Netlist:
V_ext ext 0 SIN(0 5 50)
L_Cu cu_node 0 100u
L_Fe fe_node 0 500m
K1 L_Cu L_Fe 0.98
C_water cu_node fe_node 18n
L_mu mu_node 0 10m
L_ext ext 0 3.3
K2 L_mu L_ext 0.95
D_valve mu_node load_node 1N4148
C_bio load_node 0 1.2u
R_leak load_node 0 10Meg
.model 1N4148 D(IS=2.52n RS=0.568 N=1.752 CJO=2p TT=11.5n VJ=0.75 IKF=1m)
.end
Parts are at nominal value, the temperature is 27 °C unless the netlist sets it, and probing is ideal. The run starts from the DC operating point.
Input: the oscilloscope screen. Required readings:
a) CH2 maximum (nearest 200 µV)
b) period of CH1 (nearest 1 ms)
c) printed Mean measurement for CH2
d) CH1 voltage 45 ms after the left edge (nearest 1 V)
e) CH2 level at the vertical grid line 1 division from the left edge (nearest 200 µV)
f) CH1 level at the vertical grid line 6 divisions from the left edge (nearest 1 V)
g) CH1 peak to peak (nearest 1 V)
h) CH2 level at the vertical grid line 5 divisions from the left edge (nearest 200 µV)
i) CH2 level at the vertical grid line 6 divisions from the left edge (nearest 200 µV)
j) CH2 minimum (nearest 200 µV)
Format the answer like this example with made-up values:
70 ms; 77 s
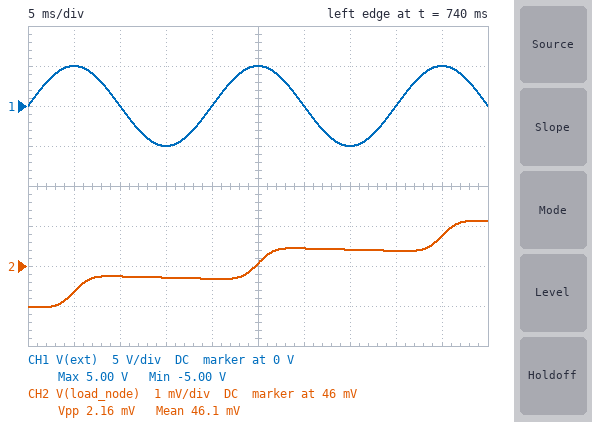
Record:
47.2 mV; 20 ms; 46.1 mV; 5 V; 45.4 mV; 0 V; 10 V; 46.0 mV; 46.4 mV; 45.0 mV
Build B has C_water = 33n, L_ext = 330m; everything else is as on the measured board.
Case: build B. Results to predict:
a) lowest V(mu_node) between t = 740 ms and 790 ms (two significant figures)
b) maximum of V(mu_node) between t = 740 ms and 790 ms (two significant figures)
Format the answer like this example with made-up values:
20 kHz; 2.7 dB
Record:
-830 mV; 830 mV
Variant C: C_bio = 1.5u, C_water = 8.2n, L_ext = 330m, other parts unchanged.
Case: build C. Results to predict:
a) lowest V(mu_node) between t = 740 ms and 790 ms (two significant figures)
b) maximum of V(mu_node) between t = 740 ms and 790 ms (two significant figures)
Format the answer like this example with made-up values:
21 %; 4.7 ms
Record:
-830 mV; 830 mV
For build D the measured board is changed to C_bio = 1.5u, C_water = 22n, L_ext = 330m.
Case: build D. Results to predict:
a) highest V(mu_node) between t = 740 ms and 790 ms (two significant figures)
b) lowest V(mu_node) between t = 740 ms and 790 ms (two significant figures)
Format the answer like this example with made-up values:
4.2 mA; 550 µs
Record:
830 mV; -830 mV
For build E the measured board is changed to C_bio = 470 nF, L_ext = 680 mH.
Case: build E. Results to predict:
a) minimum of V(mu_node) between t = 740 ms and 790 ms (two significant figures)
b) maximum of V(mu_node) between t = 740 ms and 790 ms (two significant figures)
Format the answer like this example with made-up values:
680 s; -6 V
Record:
-580 mV; 580 mV
